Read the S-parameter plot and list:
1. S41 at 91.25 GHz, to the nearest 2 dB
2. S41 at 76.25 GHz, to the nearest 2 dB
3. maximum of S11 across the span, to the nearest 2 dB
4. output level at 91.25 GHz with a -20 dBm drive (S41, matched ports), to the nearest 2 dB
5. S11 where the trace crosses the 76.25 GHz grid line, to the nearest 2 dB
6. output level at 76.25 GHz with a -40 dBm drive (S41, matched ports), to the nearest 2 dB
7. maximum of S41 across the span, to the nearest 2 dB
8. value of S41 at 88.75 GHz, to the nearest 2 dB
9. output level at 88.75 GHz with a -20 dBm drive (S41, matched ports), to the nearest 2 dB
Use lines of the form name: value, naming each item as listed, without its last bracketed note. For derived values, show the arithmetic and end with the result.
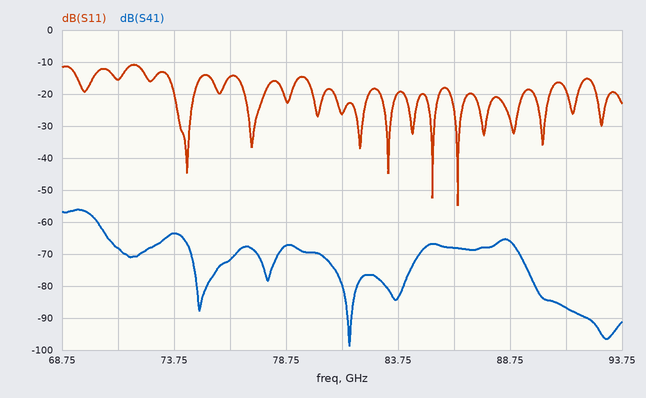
S41 at 91.25 GHz, to the nearest 2 dB: -86 dB
S41 at 76.25 GHz, to the nearest 2 dB: -72 dB
maximum of S11 across the span, to the nearest 2 dB: -10 dB
output level at 91.25 GHz with a -20 dBm drive (S41, matched ports), to the nearest 2 dB: -20 dBm + (-86 dB) = -106 dBm
S11 where the trace crosses the 76.25 GHz grid line, to the nearest 2 dB: -14 dB
output level at 76.25 GHz with a -40 dBm drive (S41, matched ports), to the nearest 2 dB: -40 dBm + (-72 dB) = -112 dBm
maximum of S41 across the span, to the nearest 2 dB: -56 dB
value of S41 at 88.75 GHz, to the nearest 2 dB: -66 dB
output level at 88.75 GHz with a -20 dBm drive (S41, matched ports), to the nearest 2 dB: -20 dBm + (-66 dB) = -86 dBm
